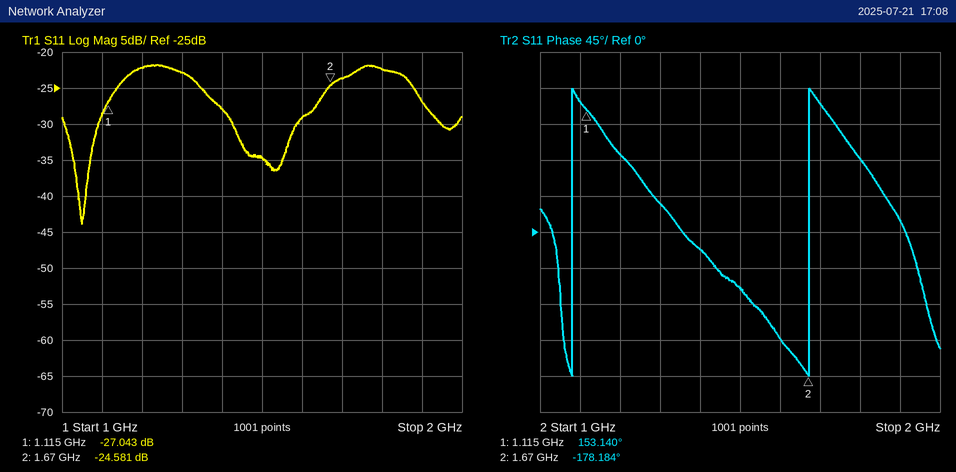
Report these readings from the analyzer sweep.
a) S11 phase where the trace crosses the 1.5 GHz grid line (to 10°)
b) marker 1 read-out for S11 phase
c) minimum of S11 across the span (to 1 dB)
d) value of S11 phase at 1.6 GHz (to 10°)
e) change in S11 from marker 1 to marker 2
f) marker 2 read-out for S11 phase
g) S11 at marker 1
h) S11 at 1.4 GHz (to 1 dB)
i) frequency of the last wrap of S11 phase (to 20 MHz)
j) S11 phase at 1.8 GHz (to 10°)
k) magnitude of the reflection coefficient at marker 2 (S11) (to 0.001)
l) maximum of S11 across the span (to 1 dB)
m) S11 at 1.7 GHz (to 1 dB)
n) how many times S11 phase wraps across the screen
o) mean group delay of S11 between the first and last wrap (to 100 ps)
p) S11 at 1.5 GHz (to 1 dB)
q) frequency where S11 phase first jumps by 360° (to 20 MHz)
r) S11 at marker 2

-70°
153.140°
-44 dB
-130°
2.462 dB
-178.184°
-27.043 dB
-28 dB
1.68 GHz
90°
0.059
-22 dB
-24 dB
2
1.7 ns
-35 dB
1.08 GHz
-24.581 dB
